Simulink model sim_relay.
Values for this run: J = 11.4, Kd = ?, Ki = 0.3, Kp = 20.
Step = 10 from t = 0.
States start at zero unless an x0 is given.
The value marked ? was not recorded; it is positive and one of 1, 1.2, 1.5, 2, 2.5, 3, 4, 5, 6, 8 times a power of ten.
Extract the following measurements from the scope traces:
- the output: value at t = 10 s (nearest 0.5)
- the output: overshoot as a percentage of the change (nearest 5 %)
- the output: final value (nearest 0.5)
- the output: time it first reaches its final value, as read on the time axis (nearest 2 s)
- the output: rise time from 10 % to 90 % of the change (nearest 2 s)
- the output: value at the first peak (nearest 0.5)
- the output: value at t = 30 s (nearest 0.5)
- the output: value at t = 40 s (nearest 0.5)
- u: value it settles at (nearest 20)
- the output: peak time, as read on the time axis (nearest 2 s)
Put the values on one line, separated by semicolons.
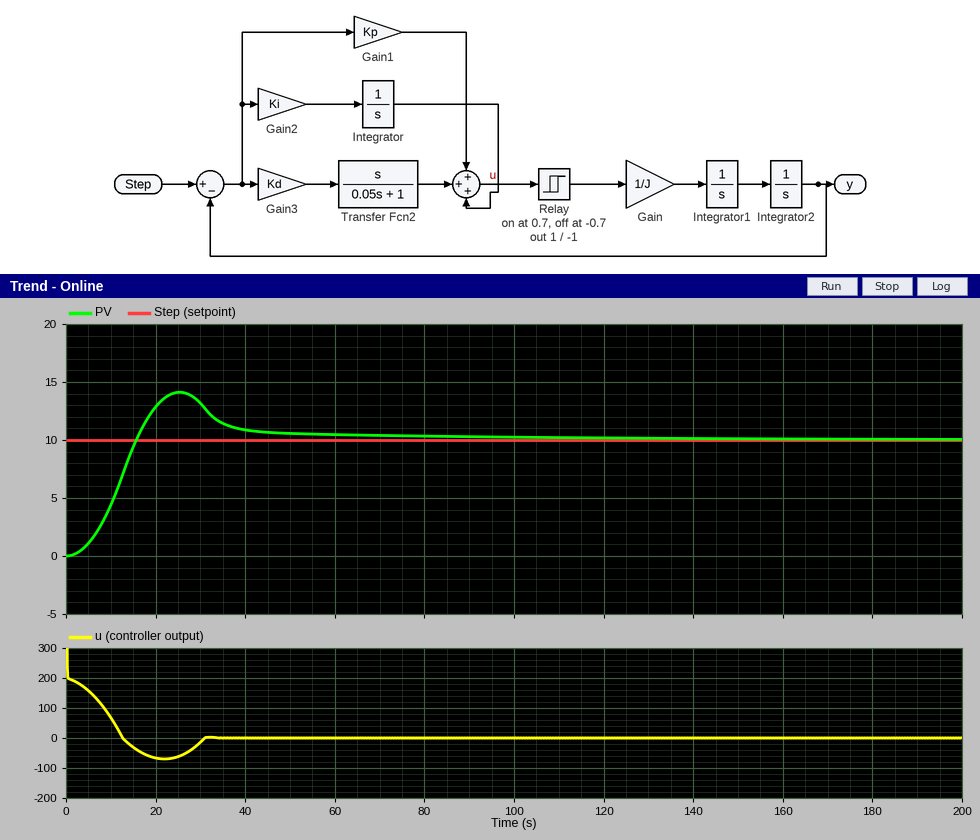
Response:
4.5; 40 %; 10.0; 16 s; 10 s; 14.0; 13.0; 11.0; 0; 26 s
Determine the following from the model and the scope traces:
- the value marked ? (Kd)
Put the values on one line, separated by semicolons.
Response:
80
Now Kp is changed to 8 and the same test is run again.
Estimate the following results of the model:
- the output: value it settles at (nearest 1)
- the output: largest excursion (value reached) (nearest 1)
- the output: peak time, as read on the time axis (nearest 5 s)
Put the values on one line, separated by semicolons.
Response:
10; 13; 35 s
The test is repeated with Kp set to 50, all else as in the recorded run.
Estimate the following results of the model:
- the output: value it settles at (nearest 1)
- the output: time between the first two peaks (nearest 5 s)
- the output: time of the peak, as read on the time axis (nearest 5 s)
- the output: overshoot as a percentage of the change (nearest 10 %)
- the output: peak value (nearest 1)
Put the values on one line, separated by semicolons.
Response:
10; 40 s; 30 s; 70 %; 17
